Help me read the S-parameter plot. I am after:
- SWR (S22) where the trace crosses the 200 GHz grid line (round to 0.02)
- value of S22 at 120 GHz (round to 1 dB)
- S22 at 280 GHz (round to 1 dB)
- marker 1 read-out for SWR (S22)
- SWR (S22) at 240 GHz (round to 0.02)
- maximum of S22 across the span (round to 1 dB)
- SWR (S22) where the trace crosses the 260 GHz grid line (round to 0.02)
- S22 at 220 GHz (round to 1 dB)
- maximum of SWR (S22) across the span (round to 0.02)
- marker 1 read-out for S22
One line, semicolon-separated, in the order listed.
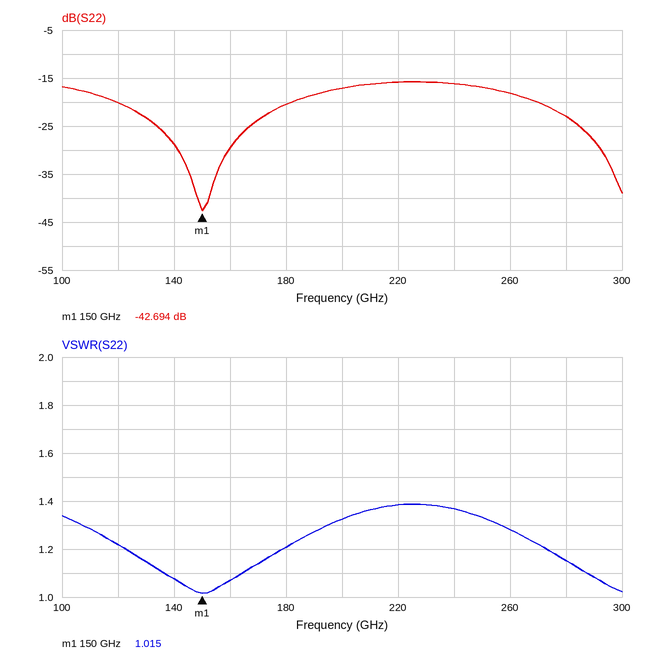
1.32; -20 dB; -23 dB; 1.015; 1.36; -16 dB; 1.28; -16 dB; 1.38; -42.694 dB
